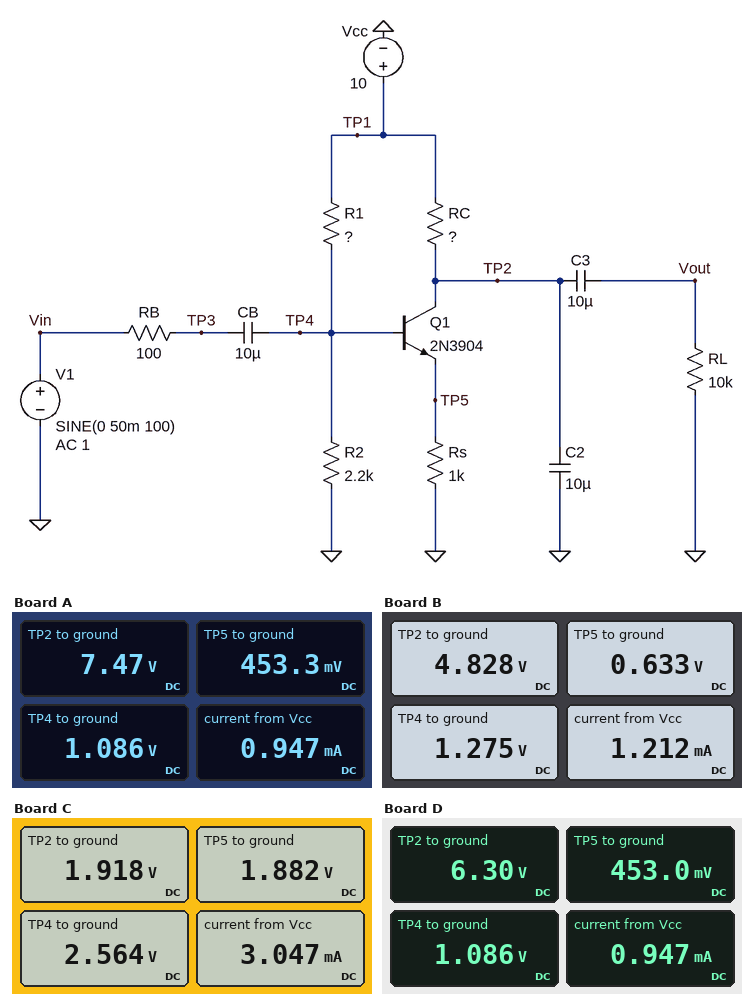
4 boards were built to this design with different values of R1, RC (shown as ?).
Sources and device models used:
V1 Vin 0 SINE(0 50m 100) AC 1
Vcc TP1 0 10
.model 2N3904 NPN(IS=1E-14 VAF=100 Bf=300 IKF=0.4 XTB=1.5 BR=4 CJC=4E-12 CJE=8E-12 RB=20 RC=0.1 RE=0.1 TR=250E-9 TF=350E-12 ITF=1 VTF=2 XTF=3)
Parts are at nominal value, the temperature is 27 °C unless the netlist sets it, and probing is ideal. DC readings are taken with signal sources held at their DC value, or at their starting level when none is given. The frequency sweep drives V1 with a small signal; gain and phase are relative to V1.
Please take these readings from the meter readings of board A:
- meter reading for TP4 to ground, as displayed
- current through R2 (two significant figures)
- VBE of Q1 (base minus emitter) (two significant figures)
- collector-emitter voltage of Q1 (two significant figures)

1.086 V
490 µA
630 mV
7.0 V
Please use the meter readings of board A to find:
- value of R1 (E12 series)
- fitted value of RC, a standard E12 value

18 kΩ
5.6 kΩ
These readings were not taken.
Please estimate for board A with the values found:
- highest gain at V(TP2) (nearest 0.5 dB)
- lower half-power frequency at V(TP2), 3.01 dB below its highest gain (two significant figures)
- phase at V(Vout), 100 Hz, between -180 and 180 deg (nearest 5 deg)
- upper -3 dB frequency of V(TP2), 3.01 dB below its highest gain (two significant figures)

1.0 dB
2.2 Hz
100 deg
15 Hz
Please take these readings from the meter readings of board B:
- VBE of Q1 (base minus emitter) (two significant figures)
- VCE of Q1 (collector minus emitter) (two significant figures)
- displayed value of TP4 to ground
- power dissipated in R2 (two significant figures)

640 mV
4.2 V
1.275 V
740 µW
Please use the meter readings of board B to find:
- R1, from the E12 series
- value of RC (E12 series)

15 kΩ
8.2 kΩ
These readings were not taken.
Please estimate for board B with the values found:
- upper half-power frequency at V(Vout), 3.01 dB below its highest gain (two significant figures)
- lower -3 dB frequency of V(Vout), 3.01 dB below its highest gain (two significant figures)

15 Hz
2.5 Hz
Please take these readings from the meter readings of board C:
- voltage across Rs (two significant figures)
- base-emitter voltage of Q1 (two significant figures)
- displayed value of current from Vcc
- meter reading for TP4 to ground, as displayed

1.9 V
680 mV
3.047 mA
2.564 V
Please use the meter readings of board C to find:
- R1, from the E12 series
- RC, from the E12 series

5.6 kΩ
4.7 kΩ
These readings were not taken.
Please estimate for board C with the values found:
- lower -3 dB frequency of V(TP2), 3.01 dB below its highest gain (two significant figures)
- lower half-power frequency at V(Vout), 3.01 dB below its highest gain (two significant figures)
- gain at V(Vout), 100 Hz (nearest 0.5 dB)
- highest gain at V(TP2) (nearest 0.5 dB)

12 Hz
12 Hz
-10.5 dB
-9.0 dB
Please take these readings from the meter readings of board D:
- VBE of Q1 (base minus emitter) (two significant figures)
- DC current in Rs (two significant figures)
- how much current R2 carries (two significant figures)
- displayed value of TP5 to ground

630 mV
450 µA
490 µA
453.0 mV
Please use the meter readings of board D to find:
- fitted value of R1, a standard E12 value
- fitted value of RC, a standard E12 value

18 kΩ
8.2 kΩ
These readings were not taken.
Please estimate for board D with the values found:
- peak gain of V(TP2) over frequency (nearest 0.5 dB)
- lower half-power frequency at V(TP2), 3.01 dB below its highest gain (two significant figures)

1.5 dB
1.9 Hz
